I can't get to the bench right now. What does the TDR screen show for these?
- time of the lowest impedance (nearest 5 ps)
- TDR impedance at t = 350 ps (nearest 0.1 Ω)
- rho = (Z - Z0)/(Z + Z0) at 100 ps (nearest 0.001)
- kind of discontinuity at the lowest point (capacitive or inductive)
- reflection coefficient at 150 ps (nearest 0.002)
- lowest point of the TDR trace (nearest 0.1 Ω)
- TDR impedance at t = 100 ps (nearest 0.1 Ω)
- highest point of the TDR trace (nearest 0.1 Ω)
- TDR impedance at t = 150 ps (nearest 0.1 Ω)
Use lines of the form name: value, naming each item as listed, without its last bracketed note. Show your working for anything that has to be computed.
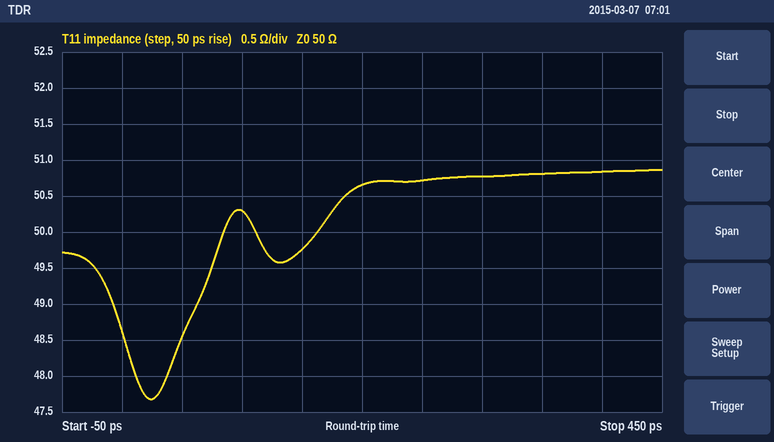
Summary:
time of the lowest impedance: 25 ps
TDR impedance at t = 350 ps: 50.8 Ω
rho = (Z - Z0)/(Z + Z0) at 100 ps: (50.3 − 50)/(50.3 + 50) ≈ +0.003
kind of discontinuity at the lowest point: capacitive
reflection coefficient at 150 ps: (49.8 − 50)/(49.8 + 50) ≈ -0.002
lowest point of the TDR trace: 47.7 Ω
TDR impedance at t = 100 ps: 50.3 Ω
highest point of the TDR trace: 50.9 Ω
TDR impedance at t = 150 ps: 49.8 Ω
